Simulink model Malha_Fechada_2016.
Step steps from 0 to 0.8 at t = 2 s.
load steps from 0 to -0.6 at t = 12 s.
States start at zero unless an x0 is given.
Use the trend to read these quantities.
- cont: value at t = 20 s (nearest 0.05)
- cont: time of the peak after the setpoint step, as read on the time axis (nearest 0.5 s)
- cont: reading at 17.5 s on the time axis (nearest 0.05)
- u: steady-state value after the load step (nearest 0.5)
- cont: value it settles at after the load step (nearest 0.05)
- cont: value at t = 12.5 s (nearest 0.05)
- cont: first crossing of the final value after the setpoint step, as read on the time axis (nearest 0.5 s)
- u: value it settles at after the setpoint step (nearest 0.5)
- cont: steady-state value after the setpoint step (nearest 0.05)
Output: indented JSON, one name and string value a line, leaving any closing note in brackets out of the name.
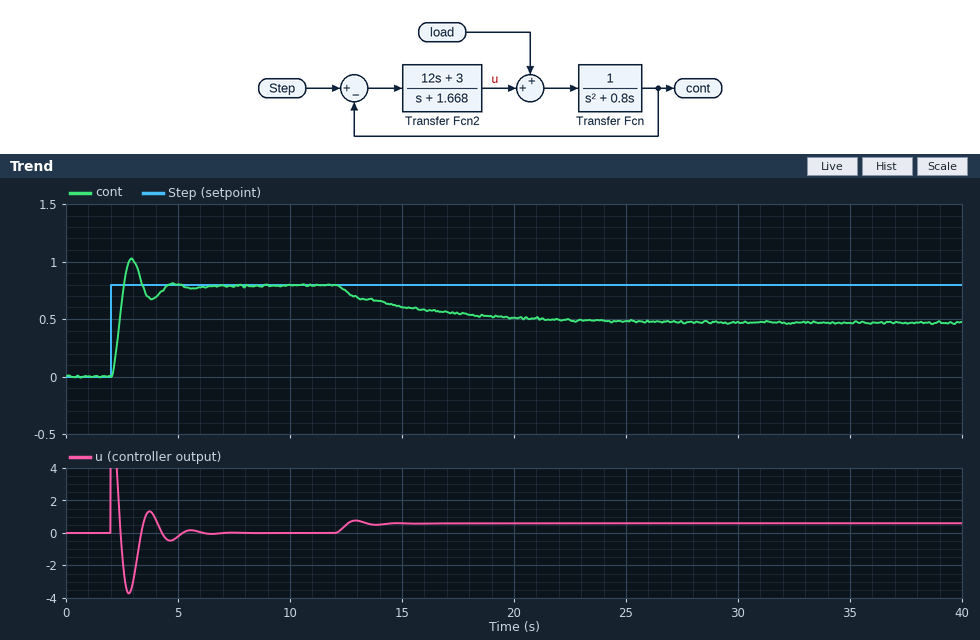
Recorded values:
{
  "cont: value at t = 20 s": "0.50",
  "cont: time of the peak after the setpoint step, as read on the time axis": "3.0 s",
  "cont: reading at 17.5 s on the time axis": "0.55",
  "u: steady-state value after the load step": "0.5",
  "cont: value it settles at after the load step": "0.45",
  "cont: value at t = 12.5 s": "0.75",
  "cont: first crossing of the final value after the setpoint step, as read on the time axis": "2.5 s",
  "u: value it settles at after the setpoint step": "0.0",
  "cont: steady-state value after the setpoint step": "0.80"
}
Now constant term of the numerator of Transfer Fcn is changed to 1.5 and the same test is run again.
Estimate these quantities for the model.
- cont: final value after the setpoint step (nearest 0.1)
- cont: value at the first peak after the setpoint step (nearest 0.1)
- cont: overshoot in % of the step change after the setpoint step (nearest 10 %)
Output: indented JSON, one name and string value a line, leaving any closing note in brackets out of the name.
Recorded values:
{
  "cont: final value after the setpoint step": "0.8",
  "cont: value at the first peak after the setpoint step": "1.1",
  "cont: overshoot in % of the step change after the setpoint step": "40 %"
}
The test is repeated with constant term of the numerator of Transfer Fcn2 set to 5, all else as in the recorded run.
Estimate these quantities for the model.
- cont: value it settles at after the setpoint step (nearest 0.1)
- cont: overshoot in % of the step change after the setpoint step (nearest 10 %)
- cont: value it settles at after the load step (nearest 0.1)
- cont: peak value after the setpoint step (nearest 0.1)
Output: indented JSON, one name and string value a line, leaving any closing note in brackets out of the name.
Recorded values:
{
  "cont: value it settles at after the setpoint step": "0.8",
  "cont: overshoot in % of the step change after the setpoint step": "30 %",
  "cont: value it settles at after the load step": "0.6",
  "cont: peak value after the setpoint step": "1.1"
}
